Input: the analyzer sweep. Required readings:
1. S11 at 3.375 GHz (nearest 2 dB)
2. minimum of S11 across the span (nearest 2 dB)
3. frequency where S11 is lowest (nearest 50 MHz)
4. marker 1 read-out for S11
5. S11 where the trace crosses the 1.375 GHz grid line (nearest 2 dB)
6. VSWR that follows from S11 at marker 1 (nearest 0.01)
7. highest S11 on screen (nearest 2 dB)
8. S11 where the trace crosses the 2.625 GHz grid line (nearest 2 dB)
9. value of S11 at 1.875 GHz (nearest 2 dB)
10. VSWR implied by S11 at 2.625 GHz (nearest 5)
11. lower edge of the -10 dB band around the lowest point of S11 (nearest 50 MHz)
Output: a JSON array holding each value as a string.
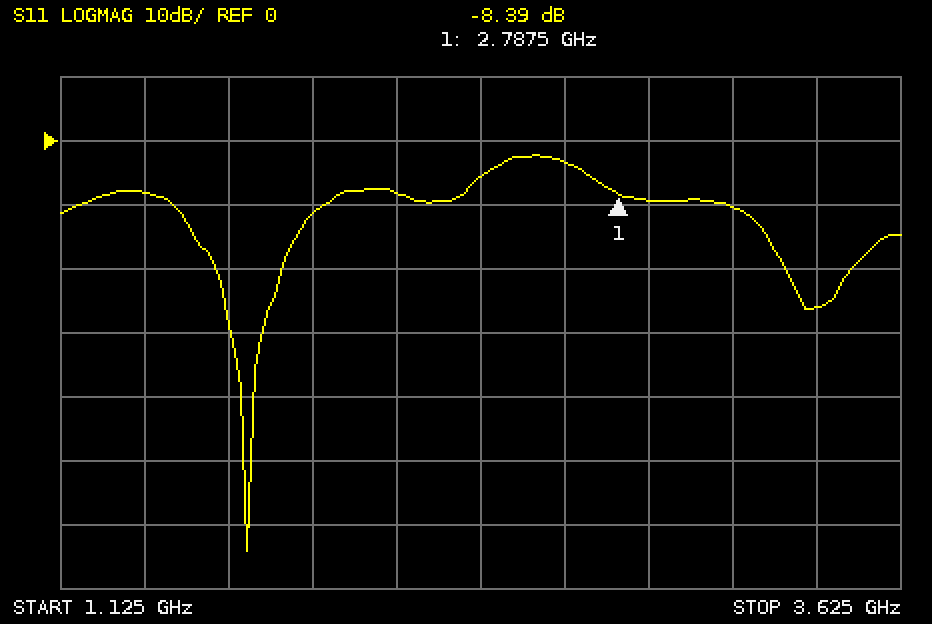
["-26 dB", "-64 dB", "1.70 GHz", "-8.39 dB", "-8 dB", "2.23", "-2 dB", "-4 dB", "-12 dB", "5", "1.45 GHz"]
